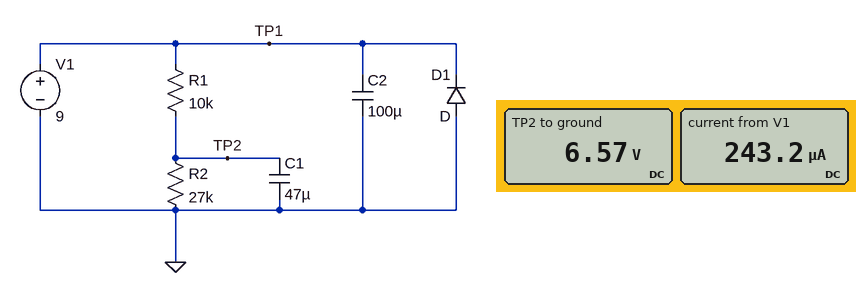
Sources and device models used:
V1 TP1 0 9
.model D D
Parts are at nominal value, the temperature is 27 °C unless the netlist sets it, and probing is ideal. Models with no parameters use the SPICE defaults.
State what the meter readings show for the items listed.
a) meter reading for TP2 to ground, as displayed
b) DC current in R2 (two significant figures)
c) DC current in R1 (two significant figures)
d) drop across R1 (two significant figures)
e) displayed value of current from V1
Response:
6.57 V
240 µA
240 µA
2.4 V
243.2 µA
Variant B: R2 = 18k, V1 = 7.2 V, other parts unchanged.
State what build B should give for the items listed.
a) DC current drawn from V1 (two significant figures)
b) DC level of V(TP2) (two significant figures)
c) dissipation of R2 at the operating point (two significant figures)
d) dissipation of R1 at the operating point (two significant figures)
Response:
260 µA
4.6 V
1.2 mW
660 µW
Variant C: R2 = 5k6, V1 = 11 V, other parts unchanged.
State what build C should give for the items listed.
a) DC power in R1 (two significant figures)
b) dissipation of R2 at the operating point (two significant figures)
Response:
5.0 mW
2.8 mW
